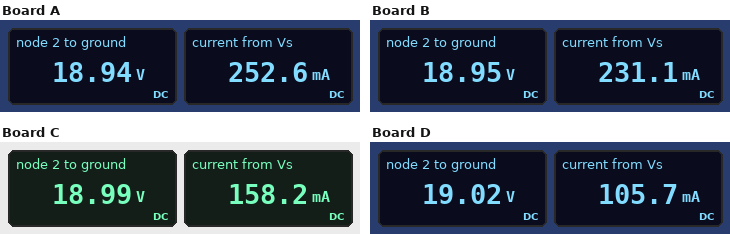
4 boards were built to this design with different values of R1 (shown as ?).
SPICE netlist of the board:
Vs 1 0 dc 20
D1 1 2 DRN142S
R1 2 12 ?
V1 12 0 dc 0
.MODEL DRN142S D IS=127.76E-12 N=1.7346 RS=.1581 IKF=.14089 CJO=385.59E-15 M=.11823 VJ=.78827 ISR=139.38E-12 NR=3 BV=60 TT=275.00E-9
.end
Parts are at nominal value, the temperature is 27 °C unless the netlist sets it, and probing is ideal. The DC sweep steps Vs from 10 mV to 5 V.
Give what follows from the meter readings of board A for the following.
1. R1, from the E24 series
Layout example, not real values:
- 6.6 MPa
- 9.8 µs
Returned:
- 75 Ω
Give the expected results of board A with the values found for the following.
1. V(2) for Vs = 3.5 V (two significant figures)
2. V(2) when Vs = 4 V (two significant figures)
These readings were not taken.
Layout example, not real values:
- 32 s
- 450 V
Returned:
- 2.6 V
- 3.1 V
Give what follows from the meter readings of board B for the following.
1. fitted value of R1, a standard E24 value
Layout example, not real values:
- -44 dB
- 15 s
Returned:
- 82 Ω
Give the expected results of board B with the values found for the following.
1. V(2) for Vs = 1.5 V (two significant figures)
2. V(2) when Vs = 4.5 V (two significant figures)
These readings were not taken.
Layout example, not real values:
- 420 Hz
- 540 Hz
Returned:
- 680 mV
- 3.6 V
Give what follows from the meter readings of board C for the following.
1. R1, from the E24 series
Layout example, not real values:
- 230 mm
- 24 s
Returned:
- 120 Ω
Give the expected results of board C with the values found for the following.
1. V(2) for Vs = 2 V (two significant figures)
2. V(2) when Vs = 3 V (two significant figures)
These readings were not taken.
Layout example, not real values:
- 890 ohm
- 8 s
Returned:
- 1.2 V
- 2.1 V
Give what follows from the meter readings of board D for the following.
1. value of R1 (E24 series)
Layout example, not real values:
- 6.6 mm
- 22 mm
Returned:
- 180 Ω
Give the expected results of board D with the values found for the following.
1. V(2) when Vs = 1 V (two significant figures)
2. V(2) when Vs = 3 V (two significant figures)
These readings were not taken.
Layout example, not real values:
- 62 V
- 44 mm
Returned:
- 270 mV
- 2.2 V
